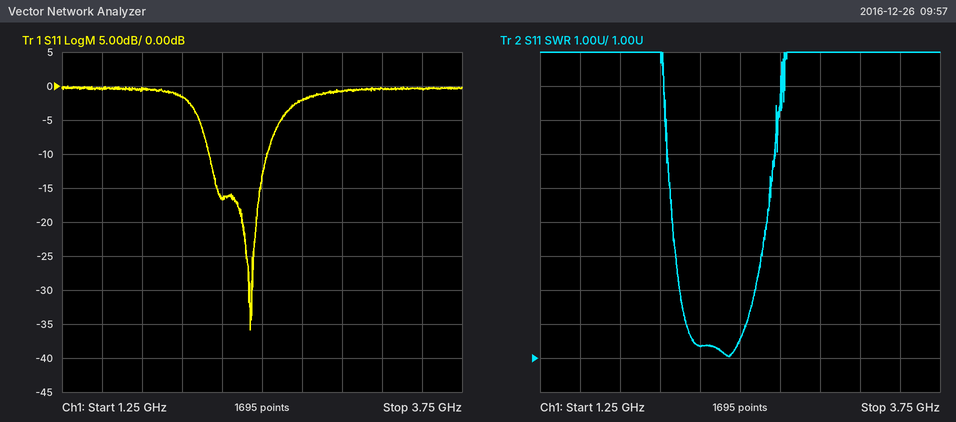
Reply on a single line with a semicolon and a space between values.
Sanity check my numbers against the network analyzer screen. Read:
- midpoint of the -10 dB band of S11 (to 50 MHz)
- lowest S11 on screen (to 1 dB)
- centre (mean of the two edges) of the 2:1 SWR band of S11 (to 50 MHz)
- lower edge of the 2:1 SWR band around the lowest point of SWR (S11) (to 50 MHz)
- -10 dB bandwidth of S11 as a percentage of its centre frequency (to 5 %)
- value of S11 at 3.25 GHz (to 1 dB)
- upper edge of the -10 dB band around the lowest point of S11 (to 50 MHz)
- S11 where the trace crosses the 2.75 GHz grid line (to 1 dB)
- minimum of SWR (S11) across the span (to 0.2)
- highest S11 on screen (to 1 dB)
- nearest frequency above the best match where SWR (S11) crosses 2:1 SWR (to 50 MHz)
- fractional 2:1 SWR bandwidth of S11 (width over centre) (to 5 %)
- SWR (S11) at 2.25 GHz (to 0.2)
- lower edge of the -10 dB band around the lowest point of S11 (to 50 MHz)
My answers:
2.35 GHz; -36 dB; 2.35 GHz; 2.15 GHz; 15 %; 0 dB; 2.55 GHz; -2 dB; 1.0; 0 dB; 2.55 GHz; 15 %; 1.4; 2.15 GHz
